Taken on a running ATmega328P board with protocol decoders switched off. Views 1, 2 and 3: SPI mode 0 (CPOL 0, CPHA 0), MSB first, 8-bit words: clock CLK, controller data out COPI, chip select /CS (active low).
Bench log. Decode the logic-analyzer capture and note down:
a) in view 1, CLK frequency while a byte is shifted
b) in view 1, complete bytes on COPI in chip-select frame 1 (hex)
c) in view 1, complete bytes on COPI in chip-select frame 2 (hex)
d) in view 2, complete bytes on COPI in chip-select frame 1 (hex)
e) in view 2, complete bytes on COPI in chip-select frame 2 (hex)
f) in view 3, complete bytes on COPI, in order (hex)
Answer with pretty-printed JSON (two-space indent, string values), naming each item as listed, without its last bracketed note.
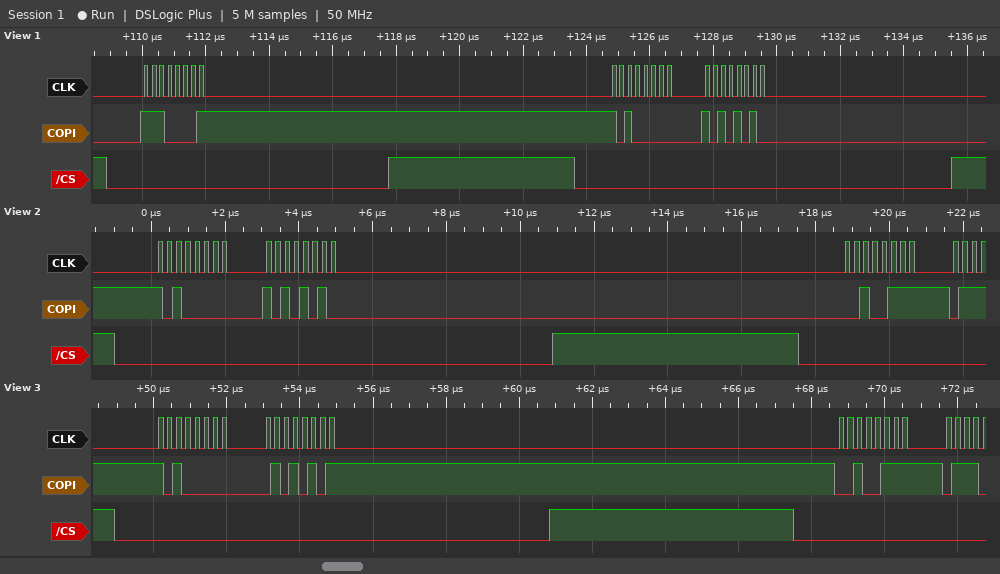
{
  "in view 1, CLK frequency while a byte is shifted": "4 MHz",
  "in view 1, complete bytes on COPI in chip-select frame 1": "E1",
  "in view 1, complete bytes on COPI in chip-select frame 2": "A0 AA",
  "in view 2, complete bytes on COPI in chip-select frame 1": "A0 AA",
  "in view 2, complete bytes on COPI in chip-select frame 2": "27",
  "in view 3, complete bytes on COPI, in order": "A0 55 27"
}
